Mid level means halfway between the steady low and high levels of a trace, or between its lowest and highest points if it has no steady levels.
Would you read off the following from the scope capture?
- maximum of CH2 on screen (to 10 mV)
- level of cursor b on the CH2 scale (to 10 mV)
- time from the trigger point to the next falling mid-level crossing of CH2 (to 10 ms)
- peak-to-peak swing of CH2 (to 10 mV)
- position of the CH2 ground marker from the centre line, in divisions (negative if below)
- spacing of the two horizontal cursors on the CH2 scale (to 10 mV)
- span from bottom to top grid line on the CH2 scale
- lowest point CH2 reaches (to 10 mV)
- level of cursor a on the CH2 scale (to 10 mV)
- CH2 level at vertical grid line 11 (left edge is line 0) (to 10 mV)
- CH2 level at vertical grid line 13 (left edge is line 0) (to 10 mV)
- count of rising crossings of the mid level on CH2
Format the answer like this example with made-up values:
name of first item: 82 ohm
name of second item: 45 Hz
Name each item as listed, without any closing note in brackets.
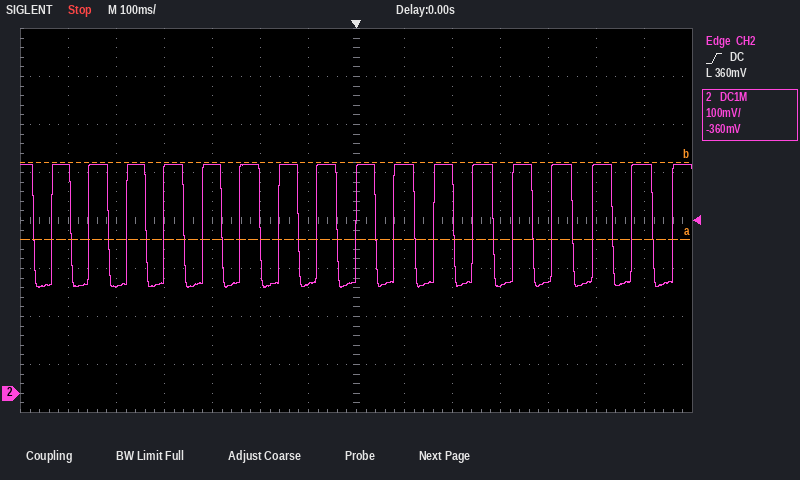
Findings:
maximum of CH2 on screen: 480 mV
level of cursor b on the CH2 scale: 480 mV
time from the trigger point to the next falling mid-level crossing of CH2: 40 ms
peak-to-peak swing of CH2: 260 mV
position of the CH2 ground marker from the centre line, in divisions: -3.6 div
spacing of the two horizontal cursors on the CH2 scale: 160 mV
span from bottom to top grid line on the CH2 scale: 800 mV
lowest point CH2 reaches: 220 mV
level of cursor a on the CH2 scale: 320 mV
CH2 level at vertical grid line 11 (left edge is line 0): 230 mV
CH2 level at vertical grid line 13 (left edge is line 0): 480 mV
count of rising crossings of the mid level on CH2: 17
